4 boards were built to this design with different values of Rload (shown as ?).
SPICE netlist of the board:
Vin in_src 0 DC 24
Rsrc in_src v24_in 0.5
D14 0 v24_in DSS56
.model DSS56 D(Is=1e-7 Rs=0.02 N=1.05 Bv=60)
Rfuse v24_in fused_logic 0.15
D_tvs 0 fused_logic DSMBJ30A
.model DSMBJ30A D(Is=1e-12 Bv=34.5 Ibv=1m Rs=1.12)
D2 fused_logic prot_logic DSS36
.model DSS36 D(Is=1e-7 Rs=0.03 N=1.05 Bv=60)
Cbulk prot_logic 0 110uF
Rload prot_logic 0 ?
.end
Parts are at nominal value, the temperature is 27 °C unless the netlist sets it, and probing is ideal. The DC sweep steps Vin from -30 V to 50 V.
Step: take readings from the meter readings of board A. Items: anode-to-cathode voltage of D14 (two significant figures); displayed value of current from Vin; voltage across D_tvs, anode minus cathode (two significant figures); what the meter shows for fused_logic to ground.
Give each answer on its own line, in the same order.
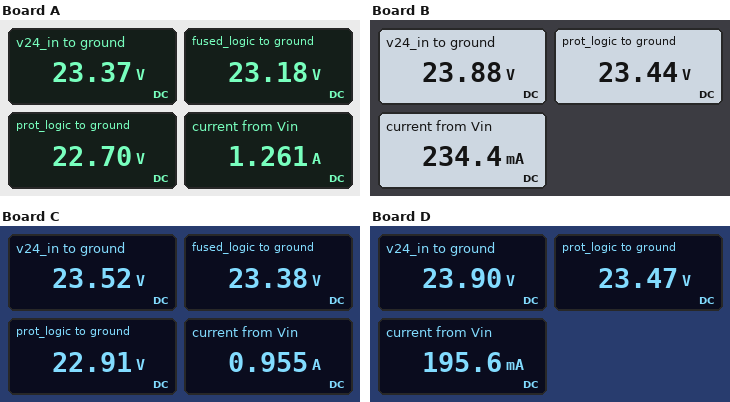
-23 V
1.261 A
-23 V
23.18 V
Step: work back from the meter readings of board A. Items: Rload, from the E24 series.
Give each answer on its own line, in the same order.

18 Ω
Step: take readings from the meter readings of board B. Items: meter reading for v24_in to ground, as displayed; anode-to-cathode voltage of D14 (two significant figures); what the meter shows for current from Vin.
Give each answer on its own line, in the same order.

23.88 V
-24 V
234.4 mA
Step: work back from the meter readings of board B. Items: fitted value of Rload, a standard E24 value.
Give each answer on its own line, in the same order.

100 Ω
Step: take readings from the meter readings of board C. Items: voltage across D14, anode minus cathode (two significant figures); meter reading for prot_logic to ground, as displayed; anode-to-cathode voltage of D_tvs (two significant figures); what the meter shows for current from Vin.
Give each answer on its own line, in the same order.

-24 V
22.91 V
-23 V
0.955 A
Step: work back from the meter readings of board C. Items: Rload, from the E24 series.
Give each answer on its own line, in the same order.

24 Ω
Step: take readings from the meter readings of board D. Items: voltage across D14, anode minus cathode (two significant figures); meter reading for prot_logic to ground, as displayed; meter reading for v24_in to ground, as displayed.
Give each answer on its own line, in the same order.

-24 V
23.47 V
23.90 V
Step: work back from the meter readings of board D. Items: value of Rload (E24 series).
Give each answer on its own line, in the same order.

120 Ω
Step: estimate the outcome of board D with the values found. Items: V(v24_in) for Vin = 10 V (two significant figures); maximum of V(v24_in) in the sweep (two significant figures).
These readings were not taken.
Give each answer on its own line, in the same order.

10 V
46 V
